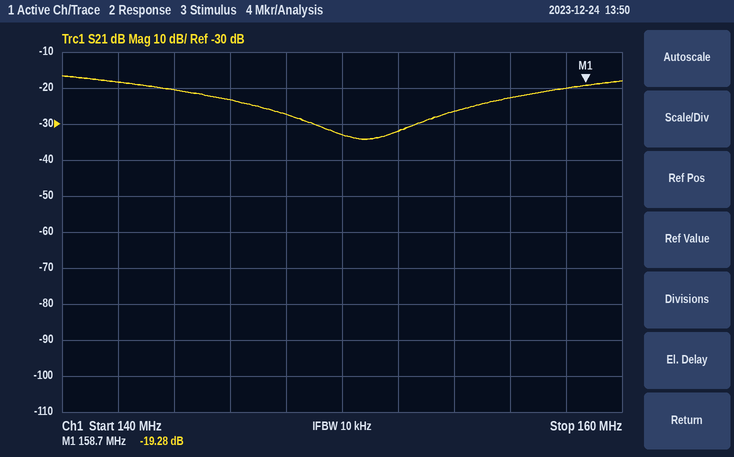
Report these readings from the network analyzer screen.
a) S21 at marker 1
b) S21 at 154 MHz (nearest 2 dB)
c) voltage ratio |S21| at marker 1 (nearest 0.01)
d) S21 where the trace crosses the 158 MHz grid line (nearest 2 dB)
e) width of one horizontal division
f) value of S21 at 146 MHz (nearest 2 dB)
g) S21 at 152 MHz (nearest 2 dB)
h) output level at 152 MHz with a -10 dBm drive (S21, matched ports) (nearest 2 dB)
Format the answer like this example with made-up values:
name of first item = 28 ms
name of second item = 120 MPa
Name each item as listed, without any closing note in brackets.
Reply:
S21 at marker 1 = -19.28 dB
S21 at 154 MHz = -26 dB
voltage ratio |S21| at marker 1 = 0.11
S21 where the trace crosses the 158 MHz grid line = -20 dB
width of one horizontal division = 2 MHz
value of S21 at 146 MHz = -24 dB
S21 at 152 MHz = -32 dB
output level at 152 MHz with a -10 dBm drive (S21, matched ports) = -42 dBm
